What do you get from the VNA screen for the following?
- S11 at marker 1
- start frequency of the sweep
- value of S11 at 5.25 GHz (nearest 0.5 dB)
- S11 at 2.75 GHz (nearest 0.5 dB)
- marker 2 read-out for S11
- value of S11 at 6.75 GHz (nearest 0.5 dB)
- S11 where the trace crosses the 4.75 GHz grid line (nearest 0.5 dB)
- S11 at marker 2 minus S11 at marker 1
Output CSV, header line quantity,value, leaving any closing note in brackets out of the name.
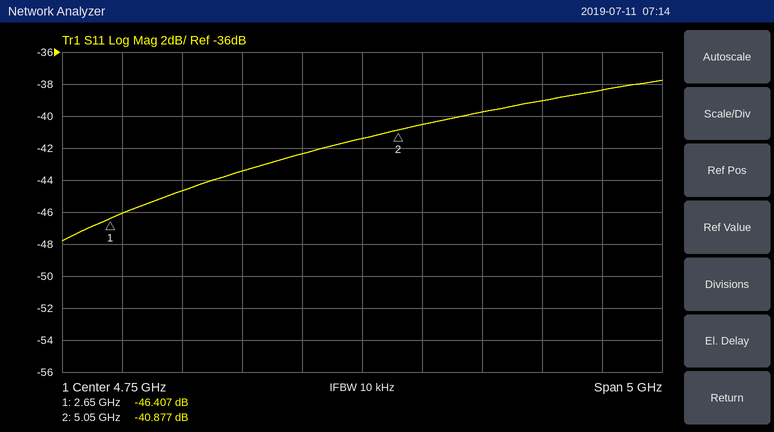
quantity,value
S11 at marker 1,-46.407 dB
start frequency of the sweep,2.25 GHz
value of S11 at 5.25 GHz,-40.5 dB
S11 at 2.75 GHz,-46.0 dB
marker 2 read-out for S11,-40.877 dB
value of S11 at 6.75 GHz,-38.5 dB
S11 where the trace crosses the 4.75 GHz grid line,-41.5 dB
S11 at marker 2 minus S11 at marker 1,5.530 dB
